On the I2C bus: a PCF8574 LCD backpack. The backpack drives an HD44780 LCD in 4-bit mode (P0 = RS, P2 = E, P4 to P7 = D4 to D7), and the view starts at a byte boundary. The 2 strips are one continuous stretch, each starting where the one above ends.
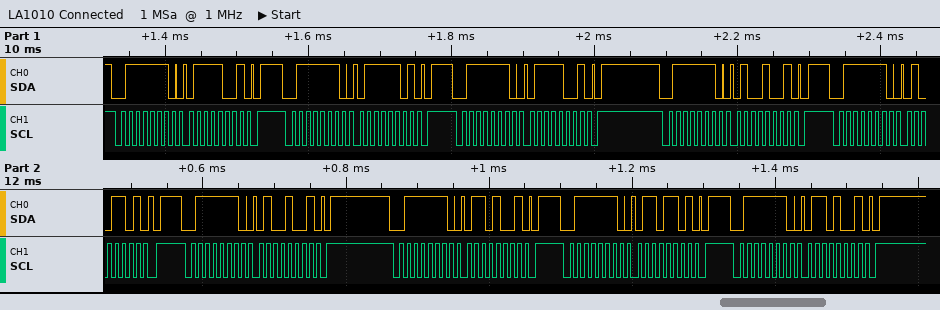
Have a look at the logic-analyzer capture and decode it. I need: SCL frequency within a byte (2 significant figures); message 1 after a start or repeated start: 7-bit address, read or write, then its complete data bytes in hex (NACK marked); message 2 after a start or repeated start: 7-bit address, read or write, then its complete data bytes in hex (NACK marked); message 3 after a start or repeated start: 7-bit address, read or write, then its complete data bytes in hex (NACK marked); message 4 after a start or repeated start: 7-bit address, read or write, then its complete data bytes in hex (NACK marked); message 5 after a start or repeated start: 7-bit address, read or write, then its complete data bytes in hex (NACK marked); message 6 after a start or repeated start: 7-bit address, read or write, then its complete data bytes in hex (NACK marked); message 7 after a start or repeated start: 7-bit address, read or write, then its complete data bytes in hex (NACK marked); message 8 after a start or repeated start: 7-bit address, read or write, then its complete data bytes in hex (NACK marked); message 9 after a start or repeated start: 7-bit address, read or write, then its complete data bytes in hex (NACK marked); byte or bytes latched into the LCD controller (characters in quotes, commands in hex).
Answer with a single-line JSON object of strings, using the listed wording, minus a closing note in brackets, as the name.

{"SCL frequency within a byte": "100 kHz", "message 1 after a start or repeated start: 7-bit address, read or write, then its complete data bytes in hex": "0x3F write: 79", "message 2 after a start or repeated start: 7-bit address, read or write, then its complete data bytes in hex": "0x3F write: 7D", "message 3 after a start or repeated start: 7-bit address, read or write, then its complete data bytes in hex": "0x3F write: 79", "message 4 after a start or repeated start: 7-bit address, read or write, then its complete data bytes in hex": "0x3F write: 49", "message 5 after a start or repeated start: 7-bit address, read or write, then its complete data bytes in hex": "0x3F write: 4D", "message 6 after a start or repeated start: 7-bit address, read or write, then its complete data bytes in hex": "0x3F write: 49", "message 7 after a start or repeated start: 7-bit address, read or write, then its complete data bytes in hex": "0x3F write: 69", "message 8 after a start or repeated start: 7-bit address, read or write, then its complete data bytes in hex": "0x3F write: 6D", "message 9 after a start or repeated start: 7-bit address, read or write, then its complete data bytes in hex": "0x3F write: 69", "byte or bytes latched into the LCD controller": "'t'"}
